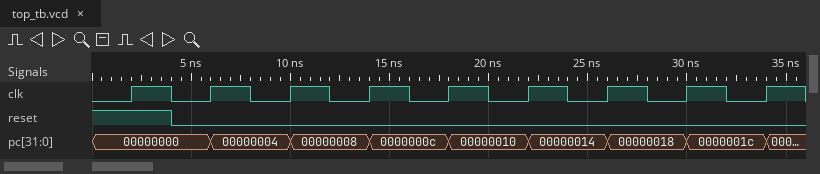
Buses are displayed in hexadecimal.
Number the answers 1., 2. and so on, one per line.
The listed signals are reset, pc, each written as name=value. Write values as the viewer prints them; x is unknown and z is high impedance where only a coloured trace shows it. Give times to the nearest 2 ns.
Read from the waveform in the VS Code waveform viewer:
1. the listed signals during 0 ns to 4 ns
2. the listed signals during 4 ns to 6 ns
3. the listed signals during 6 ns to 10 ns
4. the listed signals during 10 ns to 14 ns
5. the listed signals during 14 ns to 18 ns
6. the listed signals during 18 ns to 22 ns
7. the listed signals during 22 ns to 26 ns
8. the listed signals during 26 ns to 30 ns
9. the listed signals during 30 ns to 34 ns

1. reset=1, pc=00000000
2. reset=0, pc=00000000
3. reset=0, pc=00000004
4. reset=0, pc=00000008
5. reset=0, pc=0000000c
6. reset=0, pc=00000010
7. reset=0, pc=00000014
8. reset=0, pc=00000018
9. reset=0, pc=0000001c
